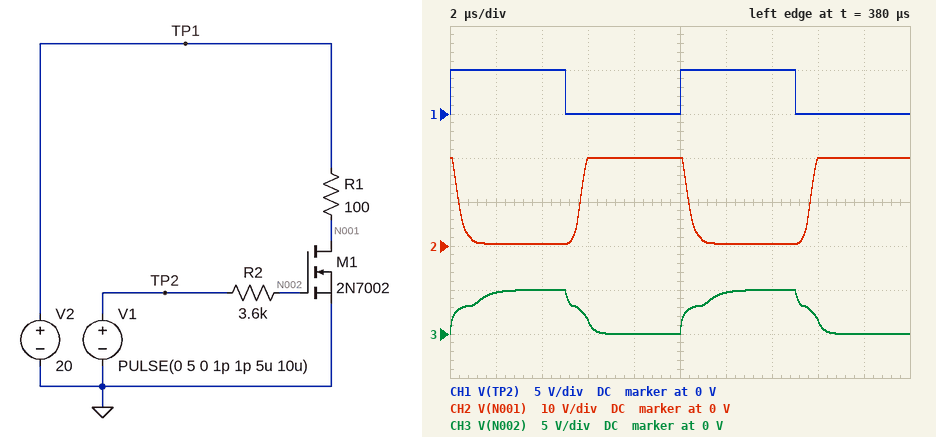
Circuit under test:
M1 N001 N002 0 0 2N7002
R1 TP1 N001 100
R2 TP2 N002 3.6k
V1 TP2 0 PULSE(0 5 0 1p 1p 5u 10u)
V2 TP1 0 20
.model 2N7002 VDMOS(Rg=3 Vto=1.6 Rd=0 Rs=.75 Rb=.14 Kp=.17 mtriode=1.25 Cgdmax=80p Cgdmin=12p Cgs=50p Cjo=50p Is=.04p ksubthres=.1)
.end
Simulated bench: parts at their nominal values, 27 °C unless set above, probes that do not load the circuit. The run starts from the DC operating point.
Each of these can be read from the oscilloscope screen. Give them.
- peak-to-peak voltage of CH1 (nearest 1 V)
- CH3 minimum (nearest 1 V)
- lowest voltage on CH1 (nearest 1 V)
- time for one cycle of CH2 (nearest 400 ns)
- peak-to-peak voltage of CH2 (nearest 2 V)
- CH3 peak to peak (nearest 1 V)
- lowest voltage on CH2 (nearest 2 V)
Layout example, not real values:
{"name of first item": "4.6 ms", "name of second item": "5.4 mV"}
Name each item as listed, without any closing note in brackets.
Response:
{"peak-to-peak voltage of CH1": "5 V", "CH3 minimum": "0 V", "lowest voltage on CH1": "0 V", "time for one cycle of CH2": "10.0 µs", "peak-to-peak voltage of CH2": "20 V", "CH3 peak to peak": "5 V", "lowest voltage on CH2": "0 V"}
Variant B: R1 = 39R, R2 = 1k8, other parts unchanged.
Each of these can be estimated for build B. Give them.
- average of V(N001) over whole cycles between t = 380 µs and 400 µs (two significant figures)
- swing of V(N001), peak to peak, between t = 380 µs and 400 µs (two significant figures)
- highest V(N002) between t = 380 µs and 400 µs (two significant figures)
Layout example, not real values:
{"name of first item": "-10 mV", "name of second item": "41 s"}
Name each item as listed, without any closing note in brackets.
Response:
{"average of V(N001) over whole cycles between t = 380 µs and 400 µs": "11 V", "swing of V(N001), peak to peak, between t = 380 µs and 400 µs": "19 V", "highest V(N002) between t = 380 µs and 400 µs": "5.0 V"}
